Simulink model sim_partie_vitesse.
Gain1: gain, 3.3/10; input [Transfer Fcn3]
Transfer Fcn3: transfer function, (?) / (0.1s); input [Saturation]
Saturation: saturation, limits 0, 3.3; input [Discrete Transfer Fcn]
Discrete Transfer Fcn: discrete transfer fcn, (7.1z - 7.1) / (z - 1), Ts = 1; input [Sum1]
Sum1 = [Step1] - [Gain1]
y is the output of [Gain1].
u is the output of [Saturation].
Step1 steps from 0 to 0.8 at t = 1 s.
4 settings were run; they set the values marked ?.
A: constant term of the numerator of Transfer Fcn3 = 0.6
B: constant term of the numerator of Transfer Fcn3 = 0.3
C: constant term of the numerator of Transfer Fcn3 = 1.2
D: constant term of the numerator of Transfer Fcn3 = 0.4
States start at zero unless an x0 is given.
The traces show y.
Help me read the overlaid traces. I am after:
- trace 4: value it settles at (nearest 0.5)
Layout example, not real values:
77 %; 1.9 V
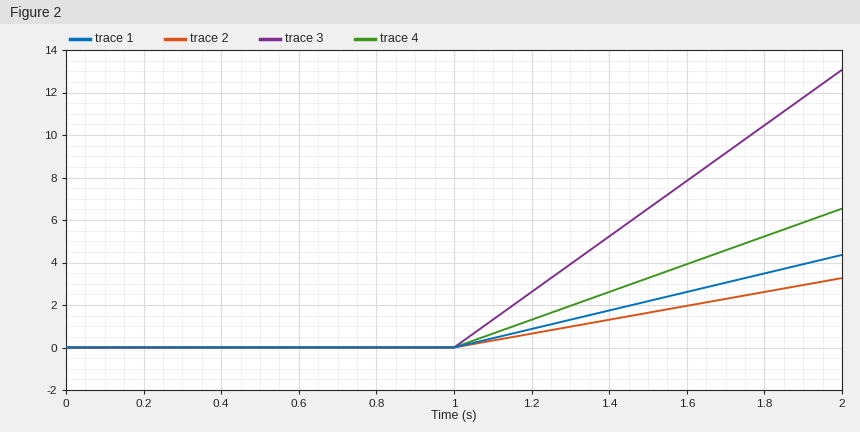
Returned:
6.5
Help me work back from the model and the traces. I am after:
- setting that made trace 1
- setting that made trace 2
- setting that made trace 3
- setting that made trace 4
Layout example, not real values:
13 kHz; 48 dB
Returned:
D; B; C; A
